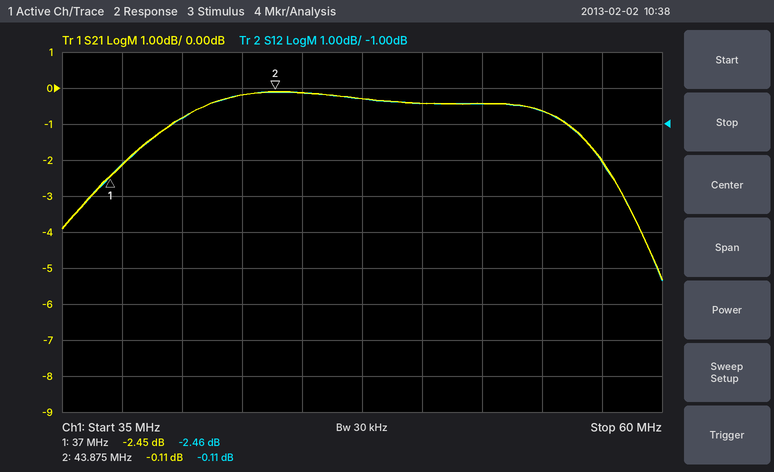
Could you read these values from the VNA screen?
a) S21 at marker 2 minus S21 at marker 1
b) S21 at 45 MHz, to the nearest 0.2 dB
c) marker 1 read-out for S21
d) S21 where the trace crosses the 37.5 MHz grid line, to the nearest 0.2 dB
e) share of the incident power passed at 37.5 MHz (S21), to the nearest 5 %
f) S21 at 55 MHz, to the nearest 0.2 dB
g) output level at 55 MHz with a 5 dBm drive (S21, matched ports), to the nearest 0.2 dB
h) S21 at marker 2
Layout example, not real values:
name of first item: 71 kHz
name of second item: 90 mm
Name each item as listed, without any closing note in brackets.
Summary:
S21 at marker 2 minus S21 at marker 1: 2.34 dB
S21 at 45 MHz, to the nearest 0.2 dB: -0.2 dB
marker 1 read-out for S21: -2.45 dB
S21 where the trace crosses the 37.5 MHz grid line, to the nearest 0.2 dB: -2.2 dB
share of the incident power passed at 37.5 MHz (S21), to the nearest 5 %: 60 %
S21 at 55 MHz, to the nearest 0.2 dB: -0.6 dB
output level at 55 MHz with a 5 dBm drive (S21, matched ports), to the nearest 0.2 dB: 4.4 dBm
S21 at marker 2: -0.11 dB
